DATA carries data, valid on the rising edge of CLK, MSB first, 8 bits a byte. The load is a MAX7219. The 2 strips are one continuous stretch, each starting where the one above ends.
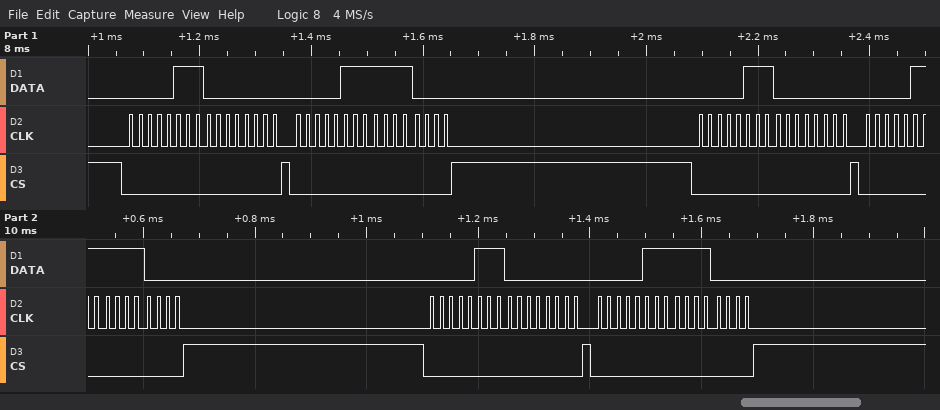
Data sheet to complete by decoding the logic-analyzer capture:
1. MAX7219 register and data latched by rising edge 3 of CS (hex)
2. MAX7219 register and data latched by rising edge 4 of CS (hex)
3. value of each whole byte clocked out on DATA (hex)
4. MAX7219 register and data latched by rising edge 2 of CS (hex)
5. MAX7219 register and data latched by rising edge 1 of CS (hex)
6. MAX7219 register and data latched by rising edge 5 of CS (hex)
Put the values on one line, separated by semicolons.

register 0x7, data 0x00; register 0x7, data 0xF0; 0x07 0x00 0x07 0xF0 0x07 0x00 0x07 0xF0 0x07 0x00 0x07 0xF0; register 0x7, data 0xF0; register 0x7, data 0x00; register 0x7, data 0x00
